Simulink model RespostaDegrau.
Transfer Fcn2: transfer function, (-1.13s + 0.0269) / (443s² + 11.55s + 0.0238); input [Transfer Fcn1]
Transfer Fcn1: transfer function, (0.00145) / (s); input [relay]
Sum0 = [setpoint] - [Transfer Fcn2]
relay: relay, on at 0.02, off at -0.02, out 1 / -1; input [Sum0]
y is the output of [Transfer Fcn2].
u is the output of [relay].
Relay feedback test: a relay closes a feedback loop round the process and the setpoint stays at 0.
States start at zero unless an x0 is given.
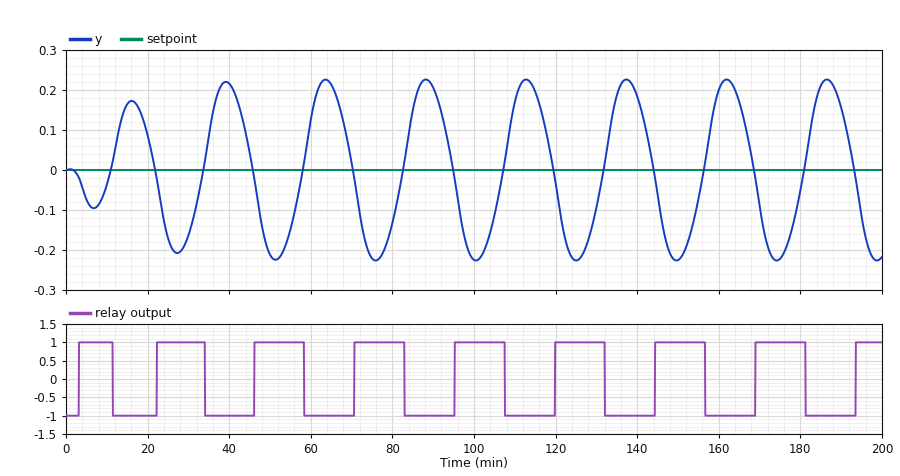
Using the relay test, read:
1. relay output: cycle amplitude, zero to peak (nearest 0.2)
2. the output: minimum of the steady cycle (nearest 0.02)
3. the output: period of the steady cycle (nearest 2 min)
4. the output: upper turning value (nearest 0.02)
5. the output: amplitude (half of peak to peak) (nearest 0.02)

1.0
-0.22
24 min
0.22
0.22
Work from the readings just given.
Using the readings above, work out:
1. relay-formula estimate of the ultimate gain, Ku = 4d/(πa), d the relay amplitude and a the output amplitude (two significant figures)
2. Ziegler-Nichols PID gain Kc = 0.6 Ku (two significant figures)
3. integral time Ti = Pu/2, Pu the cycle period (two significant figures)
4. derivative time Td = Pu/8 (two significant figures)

5.8
3.5
12 min
3.0 min
